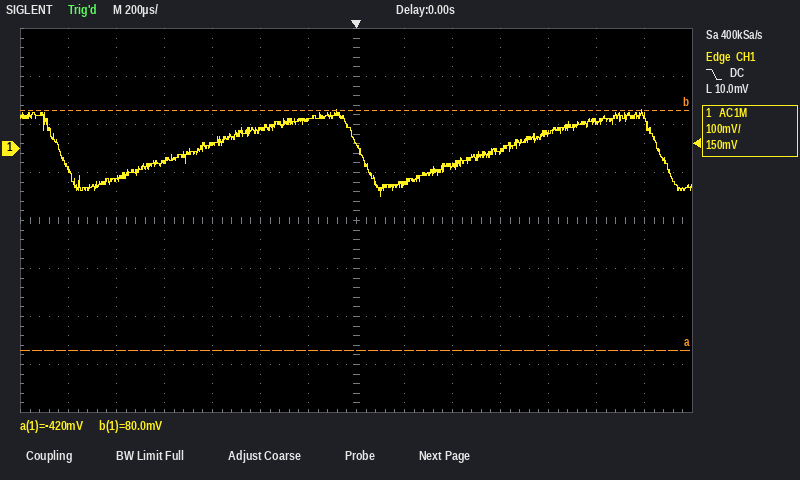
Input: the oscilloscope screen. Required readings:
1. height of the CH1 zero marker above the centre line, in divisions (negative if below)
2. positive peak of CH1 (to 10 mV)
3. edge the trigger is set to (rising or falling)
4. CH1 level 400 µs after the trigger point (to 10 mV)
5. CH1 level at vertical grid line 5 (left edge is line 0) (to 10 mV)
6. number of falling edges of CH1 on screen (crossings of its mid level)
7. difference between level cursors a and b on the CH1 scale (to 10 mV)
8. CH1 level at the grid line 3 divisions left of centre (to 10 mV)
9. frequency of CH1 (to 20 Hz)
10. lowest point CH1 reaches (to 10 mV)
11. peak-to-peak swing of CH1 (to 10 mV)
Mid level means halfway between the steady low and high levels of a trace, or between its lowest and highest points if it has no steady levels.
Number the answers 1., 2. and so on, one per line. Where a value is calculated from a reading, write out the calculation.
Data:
1. +1.5 div
2. 80 mV
3. falling
4. -40 mV
5. 40 mV
6. 3
7. 500 mV
8. 10 mV
9. 800 Hz
10. -100 mV
11. 80 mV − (-100 mV) = 180 mV
